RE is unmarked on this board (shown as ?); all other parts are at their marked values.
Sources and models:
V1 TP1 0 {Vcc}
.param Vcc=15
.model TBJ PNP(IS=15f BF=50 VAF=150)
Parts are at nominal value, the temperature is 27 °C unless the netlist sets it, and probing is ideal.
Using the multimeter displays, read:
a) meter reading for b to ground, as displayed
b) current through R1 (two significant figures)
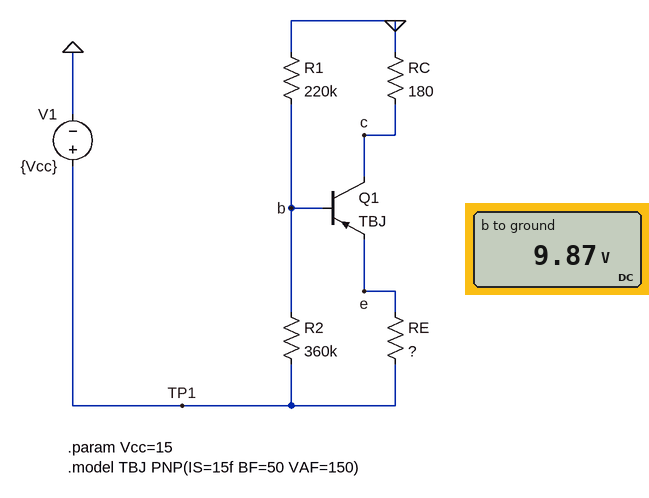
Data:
9.87 V
45 µA
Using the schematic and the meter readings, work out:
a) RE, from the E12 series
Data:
2.7 kΩ
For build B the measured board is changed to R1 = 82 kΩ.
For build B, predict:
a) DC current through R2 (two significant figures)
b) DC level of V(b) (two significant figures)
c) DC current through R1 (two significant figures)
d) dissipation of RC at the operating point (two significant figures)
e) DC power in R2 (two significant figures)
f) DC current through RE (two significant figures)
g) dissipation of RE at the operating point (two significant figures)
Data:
24 µA
6.5 V
79 µA
1.5 mW
200 µW
2.9 mA
23 mW
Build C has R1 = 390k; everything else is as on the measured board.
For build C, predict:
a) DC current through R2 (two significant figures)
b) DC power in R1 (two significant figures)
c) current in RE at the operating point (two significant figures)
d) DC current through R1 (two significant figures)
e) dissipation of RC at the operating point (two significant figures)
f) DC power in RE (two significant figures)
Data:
9.8 µA
340 µW
1.1 mA
29 µA
200 µW
3.1 mW
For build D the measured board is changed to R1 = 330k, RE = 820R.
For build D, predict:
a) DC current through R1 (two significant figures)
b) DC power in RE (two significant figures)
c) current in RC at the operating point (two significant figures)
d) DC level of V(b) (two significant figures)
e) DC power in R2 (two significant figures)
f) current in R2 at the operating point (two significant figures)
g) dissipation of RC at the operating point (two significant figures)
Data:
39 µA
2.7 mW
1.8 mA
13 V
13 µW
6.0 µA
570 µW
